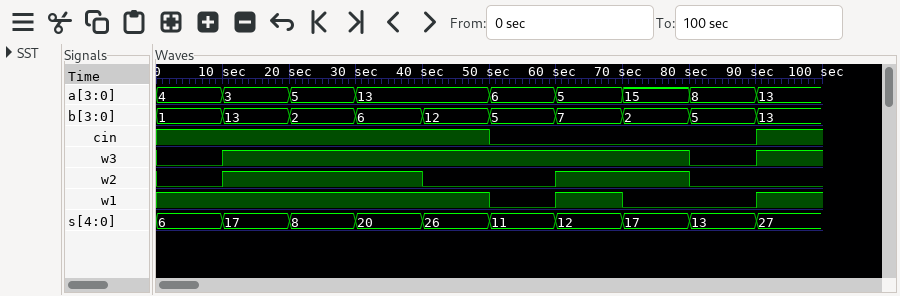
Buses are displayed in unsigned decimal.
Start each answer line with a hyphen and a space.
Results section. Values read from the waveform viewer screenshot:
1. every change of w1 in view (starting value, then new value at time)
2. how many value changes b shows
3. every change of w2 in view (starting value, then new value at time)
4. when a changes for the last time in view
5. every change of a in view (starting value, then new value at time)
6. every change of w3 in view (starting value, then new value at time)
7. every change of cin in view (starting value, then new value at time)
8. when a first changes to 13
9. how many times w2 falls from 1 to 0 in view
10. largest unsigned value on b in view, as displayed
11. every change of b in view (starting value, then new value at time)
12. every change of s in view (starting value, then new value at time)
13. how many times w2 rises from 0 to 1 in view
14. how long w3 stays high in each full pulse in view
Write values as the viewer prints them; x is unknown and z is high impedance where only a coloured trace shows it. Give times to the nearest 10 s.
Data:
- 1, 0 at 50 s, 1 at 60 s, 0 at 70 s, 1 at 90 s
- 9
- 0, 1 at 10 s, 0 at 40 s, 1 at 60 s, 0 at 80 s
- 90 s
- 4, 3 at 10 s, 5 at 20 s, 13 at 30 s, 6 at 50 s, 5 at 60 s, 15 at 70 s, 8 at 80 s, 13 at 90 s
- 0, 1 at 10 s, 0 at 80 s, 1 at 90 s
- 1, 0 at 50 s, 1 at 90 s
- 30 s
- 2
- 13
- 1, 13 at 10 s, 2 at 20 s, 6 at 30 s, 12 at 40 s, 5 at 50 s, 7 at 60 s, 2 at 70 s, 5 at 80 s, 13 at 90 s
- 6, 17 at 10 s, 8 at 20 s, 20 at 30 s, 26 at 40 s, 11 at 50 s, 12 at 60 s, 17 at 70 s, 13 at 80 s, 27 at 90 s
- 2
- 70 s
